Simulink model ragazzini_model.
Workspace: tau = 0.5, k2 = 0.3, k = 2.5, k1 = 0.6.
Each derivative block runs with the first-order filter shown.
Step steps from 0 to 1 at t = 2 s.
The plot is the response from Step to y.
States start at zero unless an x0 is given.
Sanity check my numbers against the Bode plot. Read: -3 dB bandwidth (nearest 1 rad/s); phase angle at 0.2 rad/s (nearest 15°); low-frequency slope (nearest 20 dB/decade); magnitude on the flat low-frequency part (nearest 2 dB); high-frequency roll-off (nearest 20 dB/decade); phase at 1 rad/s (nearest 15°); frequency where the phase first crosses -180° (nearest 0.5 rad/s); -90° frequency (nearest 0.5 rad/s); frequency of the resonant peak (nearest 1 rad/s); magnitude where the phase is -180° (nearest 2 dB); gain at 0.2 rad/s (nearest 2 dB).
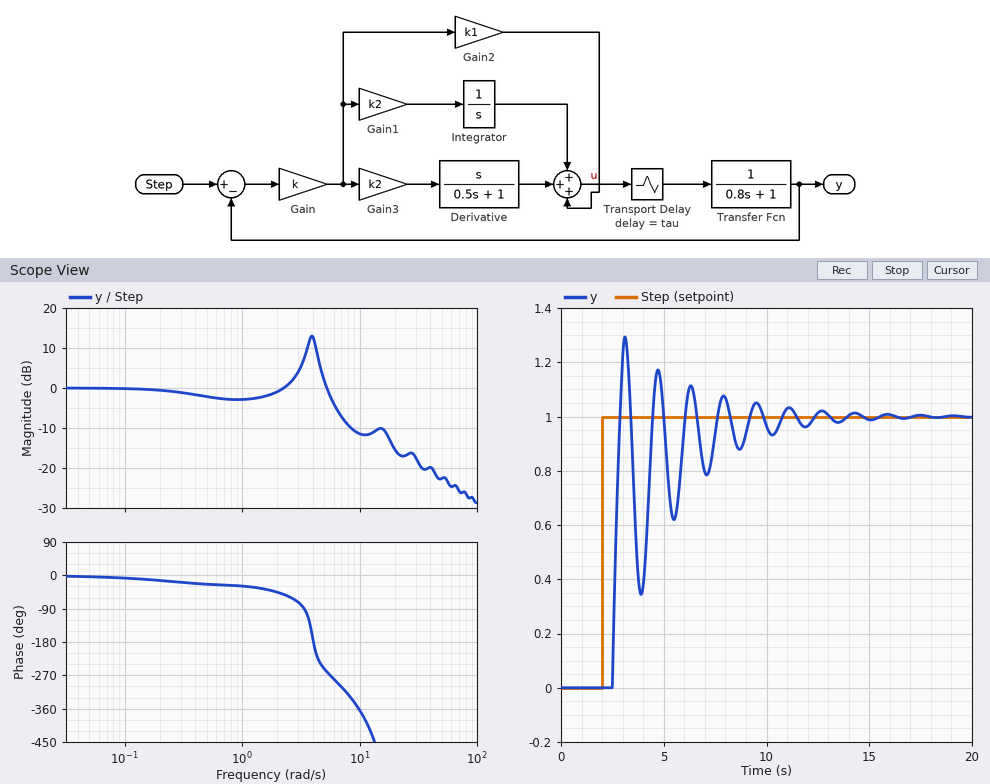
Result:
6 rad/s
-15°
0 dB/decade
0 dB
-20 dB/decade
-30°
4.0 rad/s
3.5 rad/s
4 rad/s
12 dB
0 dB
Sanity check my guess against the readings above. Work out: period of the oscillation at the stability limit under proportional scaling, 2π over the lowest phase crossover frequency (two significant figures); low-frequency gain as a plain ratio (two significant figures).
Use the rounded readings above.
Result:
1.6 s
1.0
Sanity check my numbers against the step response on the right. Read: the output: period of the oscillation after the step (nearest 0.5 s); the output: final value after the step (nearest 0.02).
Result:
1.5 s
1.00
